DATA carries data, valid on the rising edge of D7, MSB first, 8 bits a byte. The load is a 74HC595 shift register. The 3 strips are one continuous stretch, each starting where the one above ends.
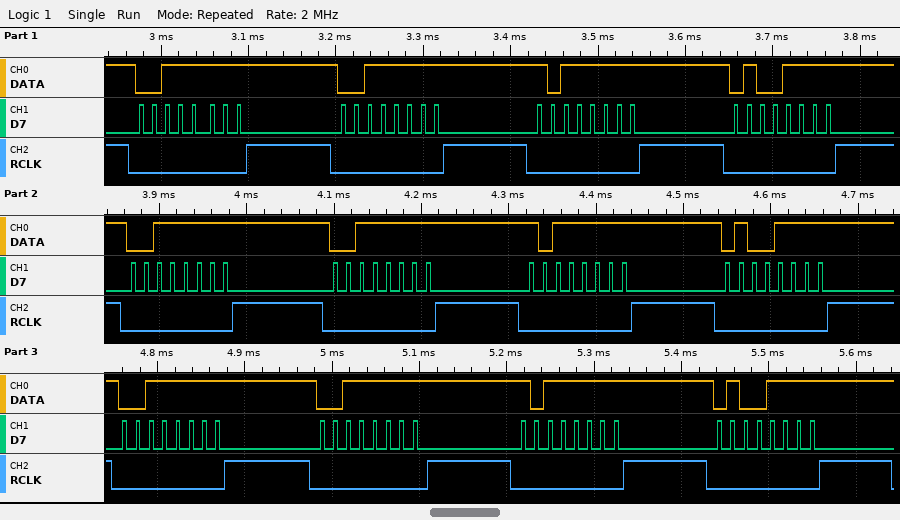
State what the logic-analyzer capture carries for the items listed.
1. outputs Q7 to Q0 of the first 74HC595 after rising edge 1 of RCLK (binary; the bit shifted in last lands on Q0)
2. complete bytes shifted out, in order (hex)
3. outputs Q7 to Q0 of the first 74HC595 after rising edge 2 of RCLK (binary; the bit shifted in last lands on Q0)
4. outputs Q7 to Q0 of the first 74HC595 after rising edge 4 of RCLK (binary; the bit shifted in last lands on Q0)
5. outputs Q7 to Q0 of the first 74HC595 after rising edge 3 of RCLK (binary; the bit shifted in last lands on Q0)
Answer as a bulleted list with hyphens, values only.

- 00111111
- 0x3F 0x3F 0xBF 0x4F 0x3F 0x3F 0xBF 0x4F 0x3F 0x3F 0xBF 0x4F
- 00111111
- 01001111
- 10111111
